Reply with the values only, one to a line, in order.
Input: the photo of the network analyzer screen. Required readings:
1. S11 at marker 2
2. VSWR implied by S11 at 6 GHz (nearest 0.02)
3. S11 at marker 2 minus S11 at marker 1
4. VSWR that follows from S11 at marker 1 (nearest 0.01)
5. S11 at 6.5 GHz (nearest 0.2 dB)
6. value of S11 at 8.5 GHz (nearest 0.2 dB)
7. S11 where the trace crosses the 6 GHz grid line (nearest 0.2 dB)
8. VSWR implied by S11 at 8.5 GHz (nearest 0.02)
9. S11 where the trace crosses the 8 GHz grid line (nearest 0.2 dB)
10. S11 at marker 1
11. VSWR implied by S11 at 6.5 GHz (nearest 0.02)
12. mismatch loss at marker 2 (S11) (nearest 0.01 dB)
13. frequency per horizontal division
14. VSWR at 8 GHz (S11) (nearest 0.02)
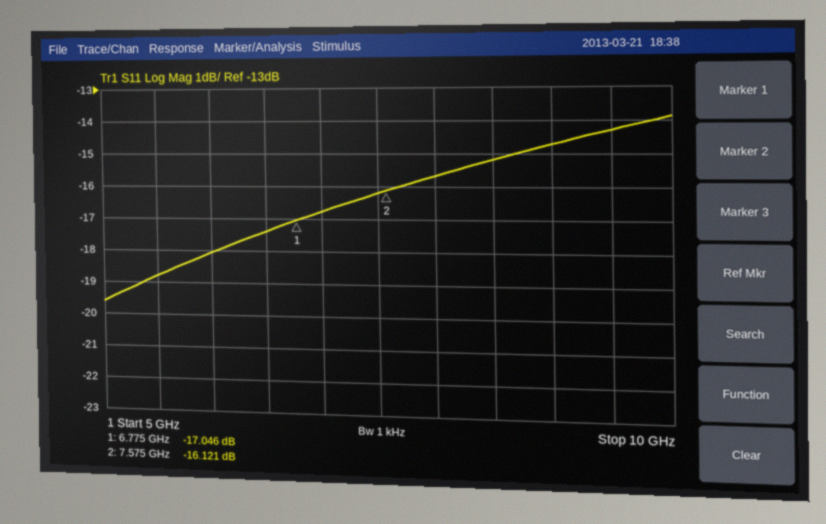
-16.121 dB
1.28
0.925 dB
1.33
-17.4 dB
-15.2 dB
-18.0 dB
1.42
-15.6 dB
-17.046 dB
1.32
0.11 dB
500 MHz
1.40
